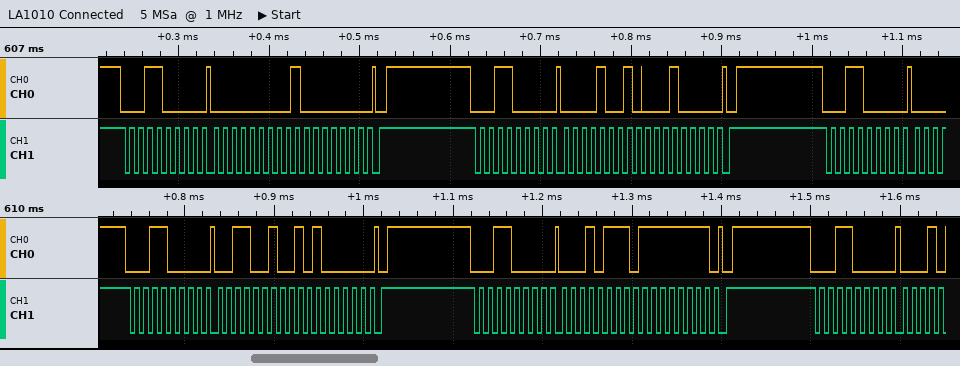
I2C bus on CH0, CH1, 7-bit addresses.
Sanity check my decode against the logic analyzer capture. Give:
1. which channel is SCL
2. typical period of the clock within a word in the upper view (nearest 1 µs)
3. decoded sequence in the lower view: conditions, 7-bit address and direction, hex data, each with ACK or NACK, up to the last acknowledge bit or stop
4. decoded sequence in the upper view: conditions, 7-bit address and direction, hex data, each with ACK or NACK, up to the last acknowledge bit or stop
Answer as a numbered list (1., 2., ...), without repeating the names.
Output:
1. CH1
2. 10 µs
3. start, address 18 write ACK, 32 ACK, A0 ACK, stop, start, address 18 write ACK, 17 ACK, FF ACK, stop, start, address 18 write ACK
4. start, address 18 write ACK, 00 ACK, 80 ACK, stop, start, address 18 write ACK, 09 ACK, 10 ACK, stop, start, address 18 write ACK
